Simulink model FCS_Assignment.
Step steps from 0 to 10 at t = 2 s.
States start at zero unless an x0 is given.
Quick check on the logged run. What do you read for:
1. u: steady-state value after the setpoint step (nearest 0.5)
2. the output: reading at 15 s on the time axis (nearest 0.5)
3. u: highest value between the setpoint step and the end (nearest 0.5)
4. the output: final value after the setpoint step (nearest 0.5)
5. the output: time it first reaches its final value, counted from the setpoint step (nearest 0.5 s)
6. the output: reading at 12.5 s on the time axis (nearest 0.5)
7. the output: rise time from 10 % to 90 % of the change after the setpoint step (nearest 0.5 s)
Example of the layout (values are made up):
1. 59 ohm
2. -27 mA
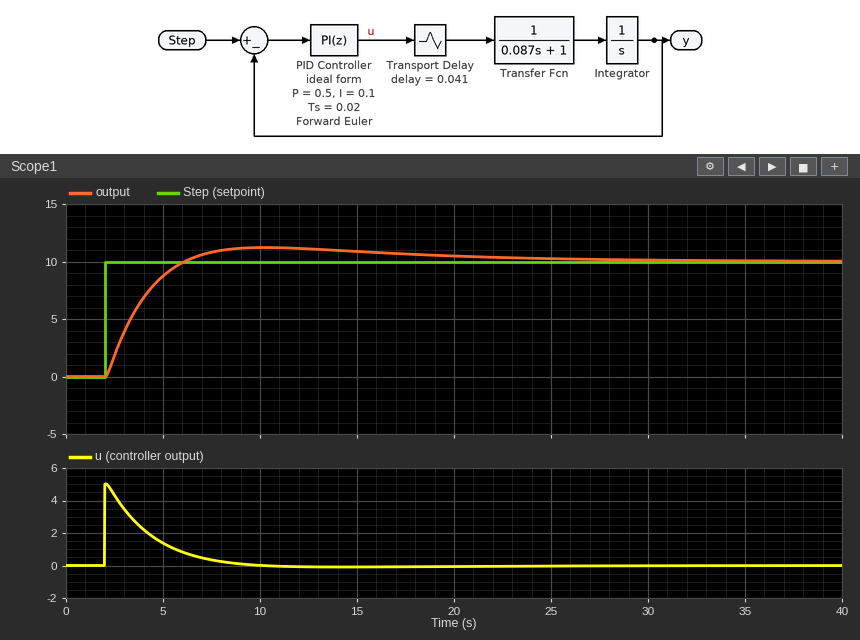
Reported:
1. 0.0
2. 11.0
3. 5.0
4. 10.0
5. 4.0 s
6. 11.0
7. 3.0 s
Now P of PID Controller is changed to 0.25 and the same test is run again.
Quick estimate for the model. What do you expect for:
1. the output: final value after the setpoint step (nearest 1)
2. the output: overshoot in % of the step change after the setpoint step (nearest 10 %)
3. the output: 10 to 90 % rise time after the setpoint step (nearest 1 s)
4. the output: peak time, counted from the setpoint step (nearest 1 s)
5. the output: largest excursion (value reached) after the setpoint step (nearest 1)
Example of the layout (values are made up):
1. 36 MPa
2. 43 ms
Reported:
1. 10
2. 20 %
3. 5 s
4. 13 s
5. 12
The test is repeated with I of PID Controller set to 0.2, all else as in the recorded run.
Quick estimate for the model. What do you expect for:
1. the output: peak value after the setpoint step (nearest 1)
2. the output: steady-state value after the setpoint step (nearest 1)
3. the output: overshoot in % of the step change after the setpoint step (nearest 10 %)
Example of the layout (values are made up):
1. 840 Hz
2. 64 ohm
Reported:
1. 12
2. 10
3. 20 %
